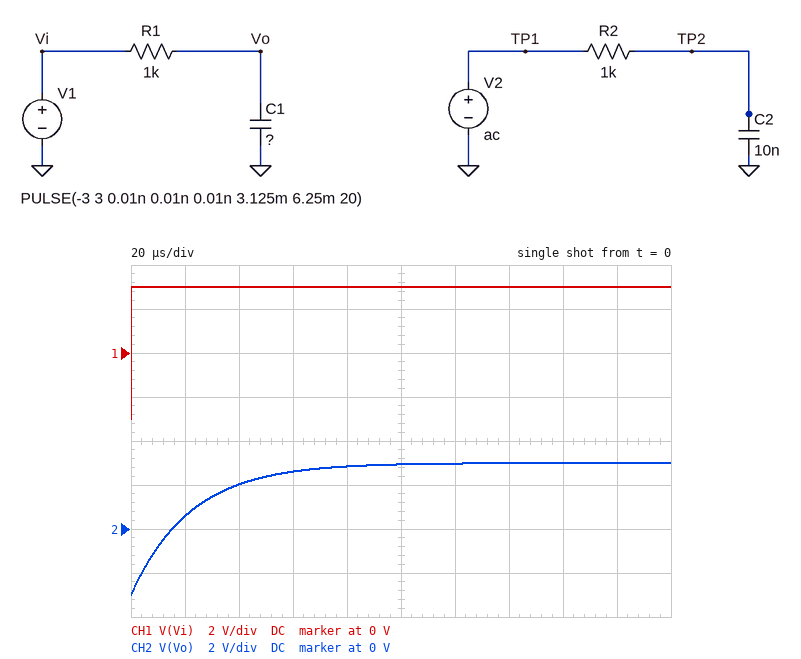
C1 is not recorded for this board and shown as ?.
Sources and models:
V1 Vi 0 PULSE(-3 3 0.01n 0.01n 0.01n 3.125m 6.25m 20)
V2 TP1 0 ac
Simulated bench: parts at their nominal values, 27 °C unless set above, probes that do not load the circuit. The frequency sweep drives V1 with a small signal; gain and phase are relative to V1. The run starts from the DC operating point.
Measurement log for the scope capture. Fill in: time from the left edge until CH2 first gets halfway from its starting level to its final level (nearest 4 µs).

16 µs
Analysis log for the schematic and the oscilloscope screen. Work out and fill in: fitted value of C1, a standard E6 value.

22 nF
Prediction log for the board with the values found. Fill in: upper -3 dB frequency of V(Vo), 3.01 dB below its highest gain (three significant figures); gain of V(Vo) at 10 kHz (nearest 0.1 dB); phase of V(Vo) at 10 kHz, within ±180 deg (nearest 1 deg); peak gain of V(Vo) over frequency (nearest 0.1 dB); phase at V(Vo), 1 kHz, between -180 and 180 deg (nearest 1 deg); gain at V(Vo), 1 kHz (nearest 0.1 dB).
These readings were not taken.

7.23 kHz
-4.6 dB
-54 deg
0 dB
-8 deg
-0.1 dB
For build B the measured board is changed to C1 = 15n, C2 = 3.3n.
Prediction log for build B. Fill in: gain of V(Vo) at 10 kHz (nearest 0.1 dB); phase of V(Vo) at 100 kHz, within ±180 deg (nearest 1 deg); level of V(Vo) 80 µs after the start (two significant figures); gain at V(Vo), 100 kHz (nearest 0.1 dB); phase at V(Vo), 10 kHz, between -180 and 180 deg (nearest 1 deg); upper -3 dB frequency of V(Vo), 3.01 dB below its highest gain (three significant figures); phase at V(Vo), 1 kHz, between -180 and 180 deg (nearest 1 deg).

-2.8 dB
-84 deg
3.0 V
-19.5 dB
-43 deg
10.6 kHz
-5 deg
